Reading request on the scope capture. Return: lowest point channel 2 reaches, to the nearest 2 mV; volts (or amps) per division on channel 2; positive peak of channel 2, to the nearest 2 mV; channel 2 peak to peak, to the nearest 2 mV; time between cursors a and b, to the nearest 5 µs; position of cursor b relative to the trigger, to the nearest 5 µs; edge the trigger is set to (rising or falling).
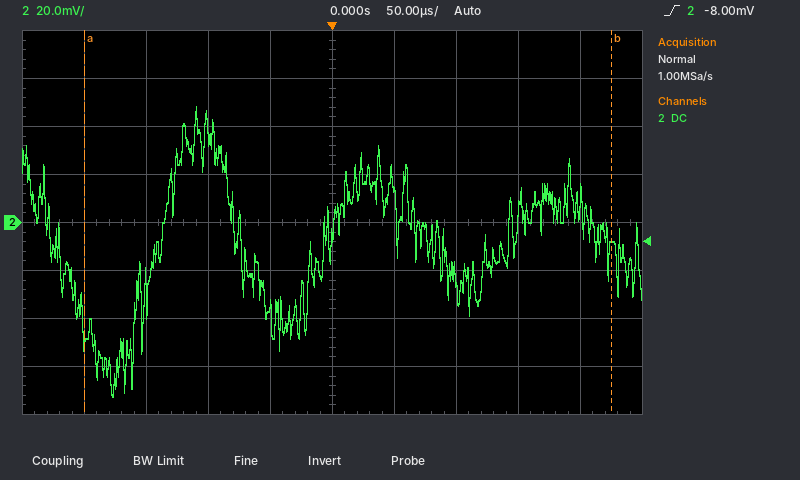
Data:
-72 mV
20 mV
48 mV
120 mV
425 µs
+225 µs
rising
